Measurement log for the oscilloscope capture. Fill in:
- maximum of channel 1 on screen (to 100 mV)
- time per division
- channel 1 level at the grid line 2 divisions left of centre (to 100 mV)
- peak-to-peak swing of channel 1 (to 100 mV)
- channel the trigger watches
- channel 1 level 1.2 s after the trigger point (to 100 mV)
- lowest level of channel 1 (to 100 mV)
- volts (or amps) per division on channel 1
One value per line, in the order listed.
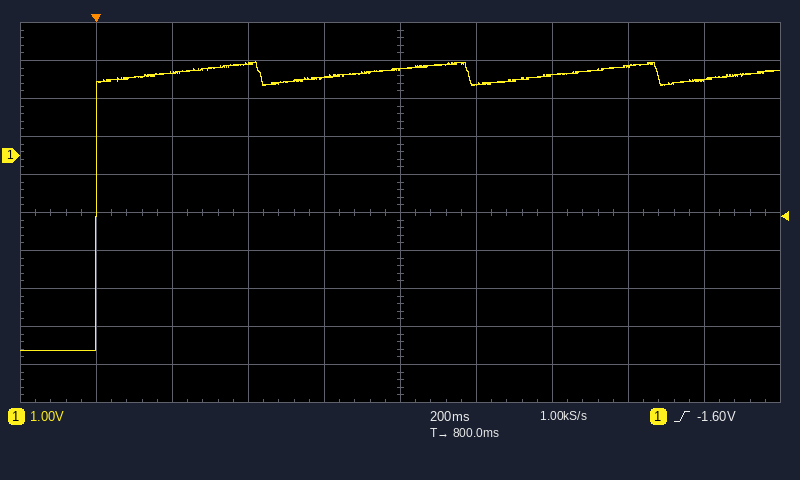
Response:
2.5 V
200 ms
2.4 V
7.6 V
channel 1
2.1 V
-5.1 V
1 V
